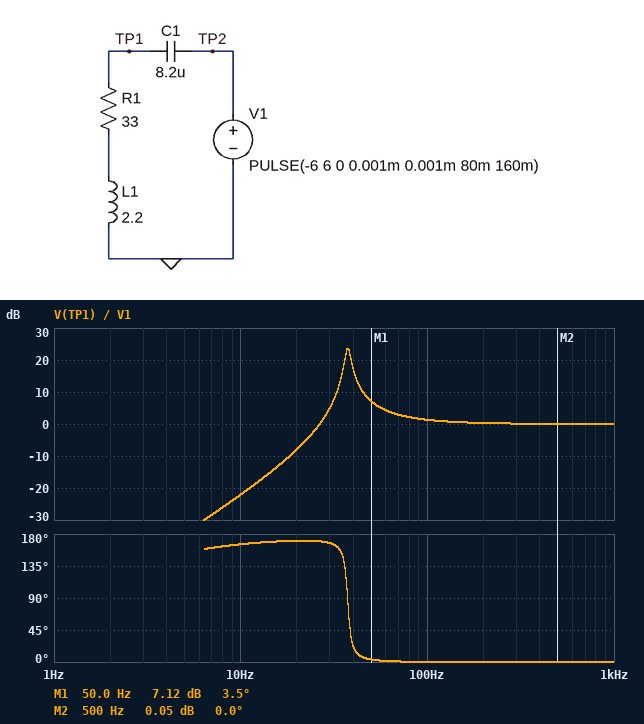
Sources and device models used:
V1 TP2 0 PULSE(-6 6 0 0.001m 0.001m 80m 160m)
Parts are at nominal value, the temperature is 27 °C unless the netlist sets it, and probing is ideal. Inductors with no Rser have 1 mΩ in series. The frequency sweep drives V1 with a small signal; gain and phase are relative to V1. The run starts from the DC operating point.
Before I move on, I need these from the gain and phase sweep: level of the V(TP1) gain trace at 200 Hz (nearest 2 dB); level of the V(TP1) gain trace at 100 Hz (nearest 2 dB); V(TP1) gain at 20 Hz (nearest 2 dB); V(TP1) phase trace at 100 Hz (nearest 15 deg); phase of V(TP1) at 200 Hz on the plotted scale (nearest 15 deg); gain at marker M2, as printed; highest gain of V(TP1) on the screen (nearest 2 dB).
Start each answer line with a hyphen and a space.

- 0 dB
- 2 dB
- -8 dB
- 0 deg
- 0 deg
- 0.05 dB
- 24 dB
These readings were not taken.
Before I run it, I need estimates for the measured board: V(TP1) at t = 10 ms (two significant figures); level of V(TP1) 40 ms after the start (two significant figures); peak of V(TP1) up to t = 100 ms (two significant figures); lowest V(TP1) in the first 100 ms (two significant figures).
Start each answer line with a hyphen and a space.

- -7.6 V
- -8.9 V
- 12 V
- -11 V
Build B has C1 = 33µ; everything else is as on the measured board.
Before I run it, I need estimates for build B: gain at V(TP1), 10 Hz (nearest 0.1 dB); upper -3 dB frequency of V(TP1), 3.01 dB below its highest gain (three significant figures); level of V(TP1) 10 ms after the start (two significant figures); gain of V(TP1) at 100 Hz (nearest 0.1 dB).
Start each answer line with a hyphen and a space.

- -7.7 dB
- 20.1 Hz
- 5.0 V
- 0.3 dB
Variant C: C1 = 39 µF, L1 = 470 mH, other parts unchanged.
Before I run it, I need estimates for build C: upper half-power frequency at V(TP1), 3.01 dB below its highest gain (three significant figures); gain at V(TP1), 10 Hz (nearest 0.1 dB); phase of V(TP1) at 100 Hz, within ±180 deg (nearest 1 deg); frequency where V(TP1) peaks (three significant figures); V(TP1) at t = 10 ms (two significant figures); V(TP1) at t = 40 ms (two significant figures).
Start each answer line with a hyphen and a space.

- 45.6 Hz
- -18.7 dB
- 1 deg
- 38.0 Hz
- -4.7 V
- -2.8 V
